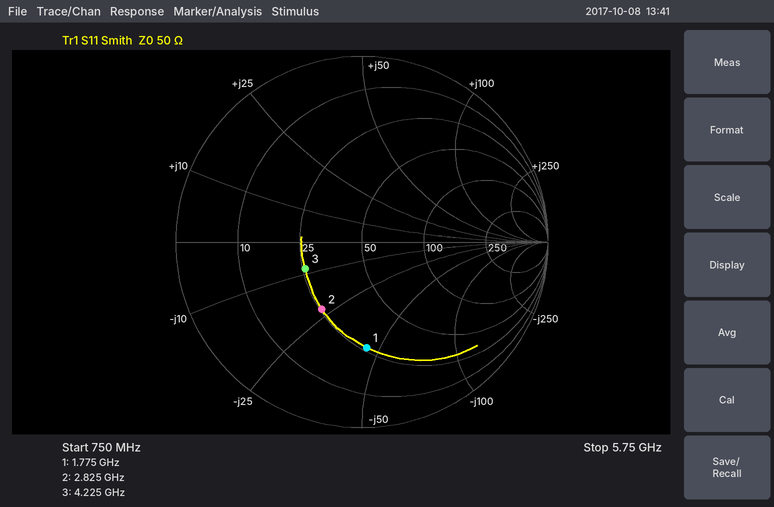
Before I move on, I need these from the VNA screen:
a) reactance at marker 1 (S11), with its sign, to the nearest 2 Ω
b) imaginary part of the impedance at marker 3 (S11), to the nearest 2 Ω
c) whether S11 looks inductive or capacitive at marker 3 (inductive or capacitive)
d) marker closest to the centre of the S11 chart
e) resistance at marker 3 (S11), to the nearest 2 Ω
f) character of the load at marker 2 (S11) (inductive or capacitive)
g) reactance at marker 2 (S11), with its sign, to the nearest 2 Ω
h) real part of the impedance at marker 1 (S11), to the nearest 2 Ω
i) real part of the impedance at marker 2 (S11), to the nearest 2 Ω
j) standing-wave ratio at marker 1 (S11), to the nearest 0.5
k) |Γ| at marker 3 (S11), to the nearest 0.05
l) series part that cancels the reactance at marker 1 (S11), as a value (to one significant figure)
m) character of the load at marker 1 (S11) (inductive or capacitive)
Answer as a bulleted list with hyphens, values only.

- -44 Ω
- -8 Ω
- capacitive
- marker 3
- 26 Ω
- capacitive
- -22 Ω
- 26 Ω
- 26 Ω
- 3.5
- 0.35
- 4 nH
- capacitive
